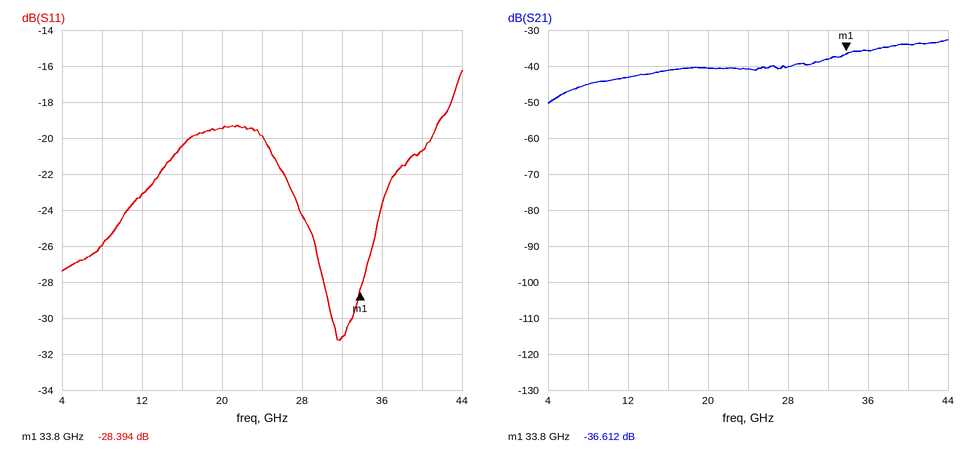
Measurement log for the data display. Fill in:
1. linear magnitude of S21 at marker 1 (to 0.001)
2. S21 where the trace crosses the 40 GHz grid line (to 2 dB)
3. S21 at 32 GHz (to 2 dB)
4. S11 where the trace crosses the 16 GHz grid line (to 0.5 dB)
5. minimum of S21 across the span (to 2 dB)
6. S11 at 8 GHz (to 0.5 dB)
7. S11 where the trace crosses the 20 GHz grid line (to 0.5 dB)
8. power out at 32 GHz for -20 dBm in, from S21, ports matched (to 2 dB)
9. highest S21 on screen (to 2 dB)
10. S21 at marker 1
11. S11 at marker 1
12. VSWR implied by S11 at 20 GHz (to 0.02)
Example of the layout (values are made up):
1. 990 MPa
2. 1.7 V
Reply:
1. 0.015
2. -34 dB
3. -38 dB
4. -20.5 dB
5. -50 dB
6. -26.0 dB
7. -19.5 dB
8. -58 dBm
9. -32 dB
10. -36.612 dB
11. -28.394 dB
12. 1.24
